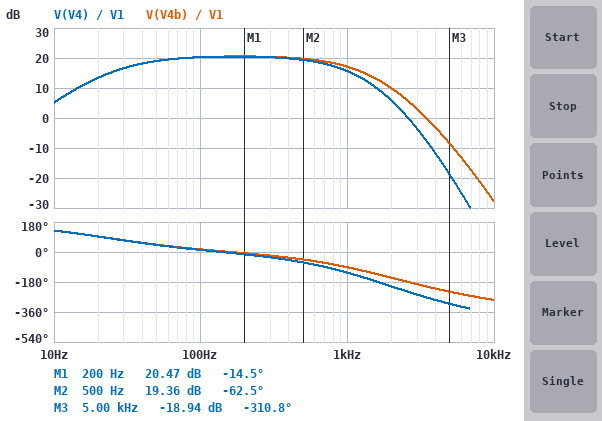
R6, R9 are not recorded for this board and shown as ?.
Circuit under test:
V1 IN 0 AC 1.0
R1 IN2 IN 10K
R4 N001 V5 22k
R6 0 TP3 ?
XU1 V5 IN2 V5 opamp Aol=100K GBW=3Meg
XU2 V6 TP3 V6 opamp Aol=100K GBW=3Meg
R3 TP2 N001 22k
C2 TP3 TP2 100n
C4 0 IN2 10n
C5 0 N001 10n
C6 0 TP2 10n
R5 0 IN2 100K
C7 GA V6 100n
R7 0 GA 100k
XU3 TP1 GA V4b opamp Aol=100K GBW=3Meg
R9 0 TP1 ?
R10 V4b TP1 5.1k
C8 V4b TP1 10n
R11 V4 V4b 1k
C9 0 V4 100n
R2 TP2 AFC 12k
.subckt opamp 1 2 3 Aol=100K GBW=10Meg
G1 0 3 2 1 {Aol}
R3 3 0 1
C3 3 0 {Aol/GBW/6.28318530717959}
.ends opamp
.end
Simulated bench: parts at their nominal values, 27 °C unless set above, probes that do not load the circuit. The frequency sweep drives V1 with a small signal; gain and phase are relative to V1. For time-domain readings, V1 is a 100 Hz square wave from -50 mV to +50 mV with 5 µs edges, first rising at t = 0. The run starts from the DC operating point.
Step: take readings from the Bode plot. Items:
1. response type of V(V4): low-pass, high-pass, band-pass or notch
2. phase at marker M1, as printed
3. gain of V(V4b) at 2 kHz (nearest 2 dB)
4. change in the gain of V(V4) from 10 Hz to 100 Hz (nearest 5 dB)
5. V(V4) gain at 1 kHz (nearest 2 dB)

band-pass
-14.5 deg
10 dB
15 dB
16 dB
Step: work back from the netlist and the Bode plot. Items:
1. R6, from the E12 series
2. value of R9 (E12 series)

2.2 kΩ
18 Ω
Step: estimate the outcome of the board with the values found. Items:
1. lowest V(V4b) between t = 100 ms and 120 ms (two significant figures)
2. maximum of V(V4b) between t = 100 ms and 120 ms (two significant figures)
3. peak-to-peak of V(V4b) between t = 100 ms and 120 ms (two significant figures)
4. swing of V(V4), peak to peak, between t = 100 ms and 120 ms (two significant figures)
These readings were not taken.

-800 mV
800 mV
1.6 V
1.6 V
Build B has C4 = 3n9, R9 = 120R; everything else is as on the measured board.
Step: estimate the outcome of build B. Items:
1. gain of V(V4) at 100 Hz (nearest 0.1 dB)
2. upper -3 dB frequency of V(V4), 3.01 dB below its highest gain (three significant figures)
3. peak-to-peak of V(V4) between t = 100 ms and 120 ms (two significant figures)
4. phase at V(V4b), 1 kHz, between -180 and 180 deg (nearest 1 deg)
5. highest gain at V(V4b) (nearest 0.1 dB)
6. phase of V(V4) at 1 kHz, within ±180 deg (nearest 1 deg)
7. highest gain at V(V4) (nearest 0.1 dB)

4.0 dB
905 Hz
240 mV
-70 deg
4.3 dB
-102 deg
4.2 dB
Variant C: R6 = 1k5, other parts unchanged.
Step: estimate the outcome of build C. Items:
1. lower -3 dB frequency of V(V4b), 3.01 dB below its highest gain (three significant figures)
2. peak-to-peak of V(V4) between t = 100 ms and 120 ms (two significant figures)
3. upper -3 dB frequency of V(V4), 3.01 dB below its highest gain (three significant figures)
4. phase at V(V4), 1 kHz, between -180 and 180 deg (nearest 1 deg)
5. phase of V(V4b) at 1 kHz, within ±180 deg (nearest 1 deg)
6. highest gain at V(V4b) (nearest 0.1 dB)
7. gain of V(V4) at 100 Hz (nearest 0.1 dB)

35.4 Hz
1.1 V
788 Hz
-121 deg
-89 deg
17.3 dB
17.0 dB
